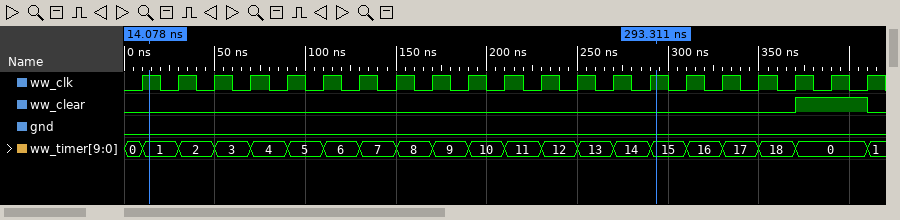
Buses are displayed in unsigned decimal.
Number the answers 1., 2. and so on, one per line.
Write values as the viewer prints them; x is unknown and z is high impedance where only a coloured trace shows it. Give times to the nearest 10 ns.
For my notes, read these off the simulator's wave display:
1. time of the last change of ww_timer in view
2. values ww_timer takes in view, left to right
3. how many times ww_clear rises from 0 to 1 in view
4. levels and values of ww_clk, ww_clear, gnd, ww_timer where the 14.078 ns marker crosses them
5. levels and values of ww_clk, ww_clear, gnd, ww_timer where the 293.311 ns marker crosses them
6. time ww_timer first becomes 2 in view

1. 410 ns
2. 0, 1, 2, 3, 4, 5, 6, 7, 8, 9, 10, 11, 12, 13, 14, 15, 16, 17, 18, 0, 1
3. 1
4. ww_clk=1, ww_clear=0, gnd=0, ww_timer=1
5. ww_clk=1, ww_clear=0, gnd=0, ww_timer=15
6. 30 ns
